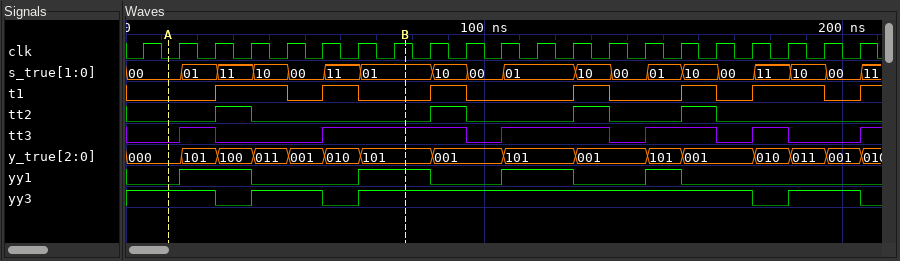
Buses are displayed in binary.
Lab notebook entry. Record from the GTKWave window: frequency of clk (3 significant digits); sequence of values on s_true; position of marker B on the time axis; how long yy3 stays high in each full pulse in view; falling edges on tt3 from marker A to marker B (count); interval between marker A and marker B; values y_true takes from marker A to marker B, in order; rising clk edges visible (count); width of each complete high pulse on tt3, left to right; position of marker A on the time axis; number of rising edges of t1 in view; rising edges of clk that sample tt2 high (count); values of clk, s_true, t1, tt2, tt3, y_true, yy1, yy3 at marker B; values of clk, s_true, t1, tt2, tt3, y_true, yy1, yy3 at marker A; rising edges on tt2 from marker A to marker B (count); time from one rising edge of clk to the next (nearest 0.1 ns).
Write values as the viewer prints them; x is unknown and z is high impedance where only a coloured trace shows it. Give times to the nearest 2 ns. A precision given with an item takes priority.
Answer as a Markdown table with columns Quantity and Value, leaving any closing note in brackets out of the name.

| Quantity | Value |
|---|---|
| frequency of clk | 100 MHz |
| sequence of values on s_true | 00, 01, 11, 10, 00, 11, 01, 10, 00, 01, 10, 00, 01, 10, 00, 11, 10, 00, 11 |
| position of marker B on the time axis | 78 ns |
| how long yy3 stays high in each full pulse in view | 20 ns, 110 ns, 20 ns |
| falling edges on tt3 from marker A to marker B | 1 |
| interval between marker A and marker B | 66 ns |
| values y_true takes from marker A to marker B, in order | 000, 101, 100, 011, 001, 010, 101 |
| rising clk edges visible | 21 |
| width of each complete high pulse on tt3, left to right | 10 ns, 40 ns, 30 ns, 20 ns, 10 ns |
| position of marker A on the time axis | 12 ns |
| number of rising edges of t1 in view | 7 |
| rising edges of clk that sample tt2 high | 4 |
| values of clk, s_true, t1, tt2, tt3, y_true, yy1, yy3 at marker B | clk=1, s_true=01, t1=0, tt2=0, tt3=1, y_true=101, yy1=1, yy3=1 |
| values of clk, s_true, t1, tt2, tt3, y_true, yy1, yy3 at marker A | clk=0, s_true=00, t1=0, tt2=0, tt3=0, y_true=000, yy1=0, yy3=1 |
| rising edges on tt2 from marker A to marker B | 1 |
| time from one rising edge of clk to the next | 10 ns |
